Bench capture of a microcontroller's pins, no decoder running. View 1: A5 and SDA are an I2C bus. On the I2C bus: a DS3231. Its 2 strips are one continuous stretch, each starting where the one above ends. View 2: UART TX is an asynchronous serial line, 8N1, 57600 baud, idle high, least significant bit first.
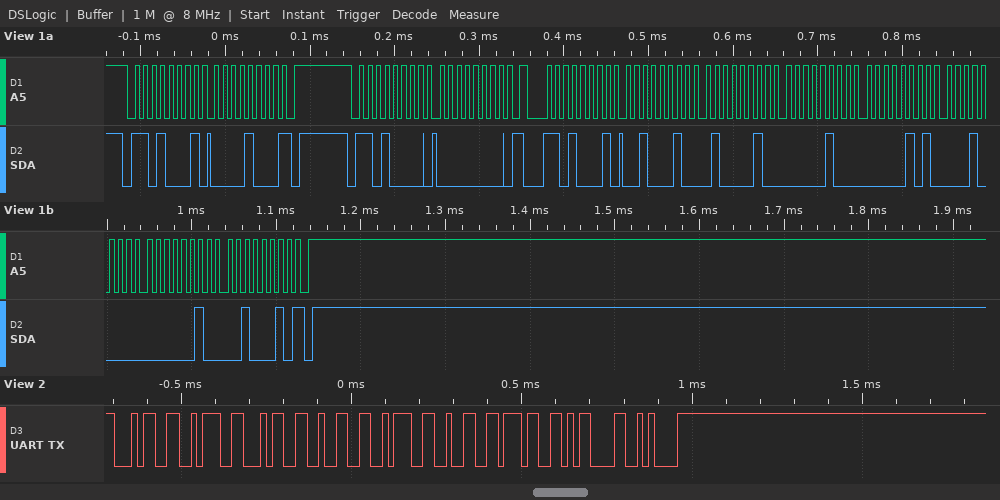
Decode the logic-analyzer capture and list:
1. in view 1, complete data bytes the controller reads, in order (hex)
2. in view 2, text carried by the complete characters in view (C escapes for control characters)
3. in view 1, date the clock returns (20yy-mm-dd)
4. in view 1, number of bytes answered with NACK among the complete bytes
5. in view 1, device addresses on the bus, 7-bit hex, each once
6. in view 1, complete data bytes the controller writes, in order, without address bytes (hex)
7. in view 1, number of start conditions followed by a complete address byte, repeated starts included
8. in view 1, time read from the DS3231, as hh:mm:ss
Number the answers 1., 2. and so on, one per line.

1. 08 22 42 04 05 10 02 22
2. "4:42:27\r\n"
3. 2022-02-10
4. 2
5. 0x68
6. 00
7. 3
8. 04:42:22
